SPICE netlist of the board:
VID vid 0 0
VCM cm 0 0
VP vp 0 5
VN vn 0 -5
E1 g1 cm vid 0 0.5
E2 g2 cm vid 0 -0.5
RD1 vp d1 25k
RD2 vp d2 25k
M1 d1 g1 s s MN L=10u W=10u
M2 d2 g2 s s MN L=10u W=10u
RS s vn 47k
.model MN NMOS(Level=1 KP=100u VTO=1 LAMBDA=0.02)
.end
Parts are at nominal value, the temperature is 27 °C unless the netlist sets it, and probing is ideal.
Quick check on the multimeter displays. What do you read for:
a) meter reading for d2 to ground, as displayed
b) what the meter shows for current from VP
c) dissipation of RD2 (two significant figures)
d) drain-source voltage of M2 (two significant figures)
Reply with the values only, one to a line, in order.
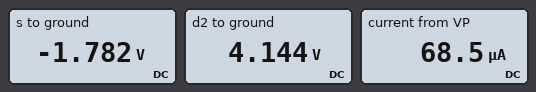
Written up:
4.144 V
68.5 µA
29 µW
5.9 V
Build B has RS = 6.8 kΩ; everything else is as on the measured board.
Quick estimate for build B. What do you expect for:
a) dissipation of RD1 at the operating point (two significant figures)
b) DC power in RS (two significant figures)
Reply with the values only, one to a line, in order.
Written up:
680 µW
740 µW
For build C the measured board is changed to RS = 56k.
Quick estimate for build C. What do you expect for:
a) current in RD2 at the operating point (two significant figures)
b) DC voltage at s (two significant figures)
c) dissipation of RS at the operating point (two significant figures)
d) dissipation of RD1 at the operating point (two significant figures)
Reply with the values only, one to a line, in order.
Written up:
29 µA
-1.7 V
190 µW
21 µW
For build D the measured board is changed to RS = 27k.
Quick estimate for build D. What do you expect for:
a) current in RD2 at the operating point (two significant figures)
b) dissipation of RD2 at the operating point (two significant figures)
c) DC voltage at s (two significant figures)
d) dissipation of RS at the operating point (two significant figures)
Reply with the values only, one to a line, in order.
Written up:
56 µA
77 µW
-2.0 V
330 µW
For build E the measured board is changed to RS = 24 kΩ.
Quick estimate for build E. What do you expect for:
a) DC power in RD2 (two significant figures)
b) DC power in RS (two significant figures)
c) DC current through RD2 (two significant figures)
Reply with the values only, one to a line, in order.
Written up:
94 µW
360 µW
61 µA
